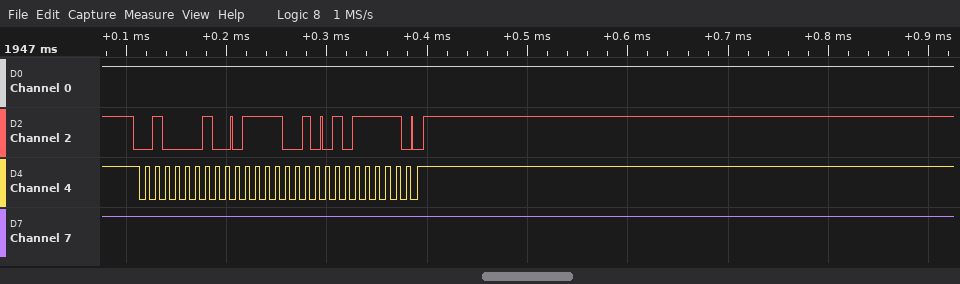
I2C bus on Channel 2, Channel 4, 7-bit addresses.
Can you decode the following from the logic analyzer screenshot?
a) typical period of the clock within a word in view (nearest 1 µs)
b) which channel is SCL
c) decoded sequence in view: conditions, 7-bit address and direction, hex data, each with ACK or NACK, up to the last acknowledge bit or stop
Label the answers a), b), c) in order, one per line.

a) 10 µs
b) Channel 4
c) start, address 21 write ACK, 79 ACK, 5F ACK, stop
